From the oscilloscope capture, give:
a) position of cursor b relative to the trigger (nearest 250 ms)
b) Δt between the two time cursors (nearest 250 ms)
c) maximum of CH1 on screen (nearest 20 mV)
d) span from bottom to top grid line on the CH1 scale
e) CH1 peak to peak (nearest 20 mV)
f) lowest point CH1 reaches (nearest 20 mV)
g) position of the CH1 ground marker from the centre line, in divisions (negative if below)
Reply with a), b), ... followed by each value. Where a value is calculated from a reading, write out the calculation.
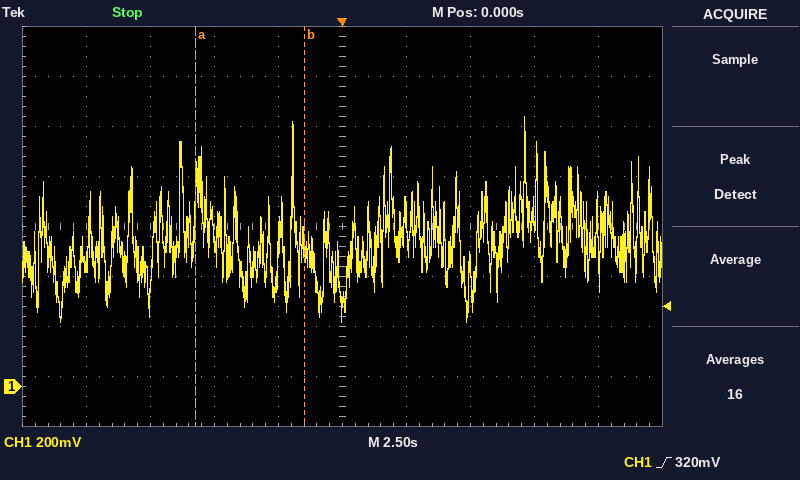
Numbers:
a) -1.50 s
b) 4.25 s
c) 1.08 V
d) 1.6 V
e) 1.08 V − (260 mV) = 820 mV
f) 260 mV
g) -3.2 div
